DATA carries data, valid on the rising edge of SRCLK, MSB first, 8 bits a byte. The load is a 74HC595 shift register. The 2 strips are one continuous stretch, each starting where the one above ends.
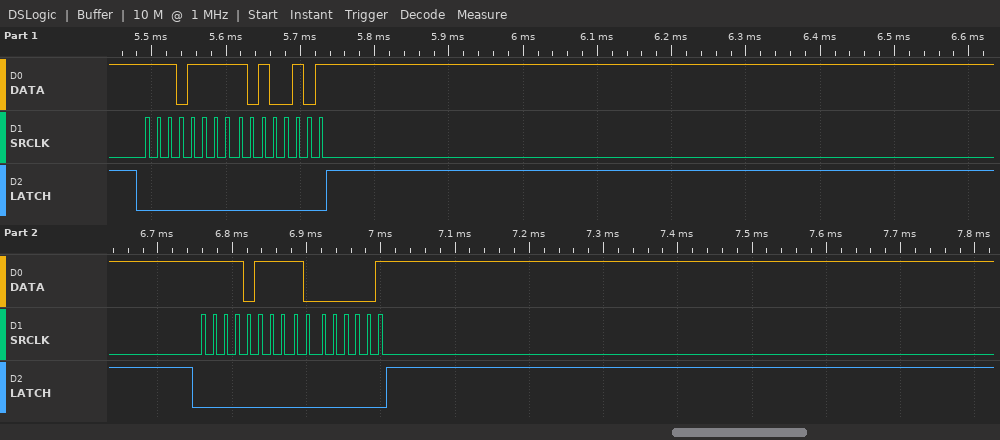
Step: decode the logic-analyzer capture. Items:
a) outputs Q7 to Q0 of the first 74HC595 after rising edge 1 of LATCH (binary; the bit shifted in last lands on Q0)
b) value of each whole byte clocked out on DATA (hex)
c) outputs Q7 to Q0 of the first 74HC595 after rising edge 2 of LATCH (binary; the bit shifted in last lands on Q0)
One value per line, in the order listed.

10100101
EF A5 F7 81
10000001
